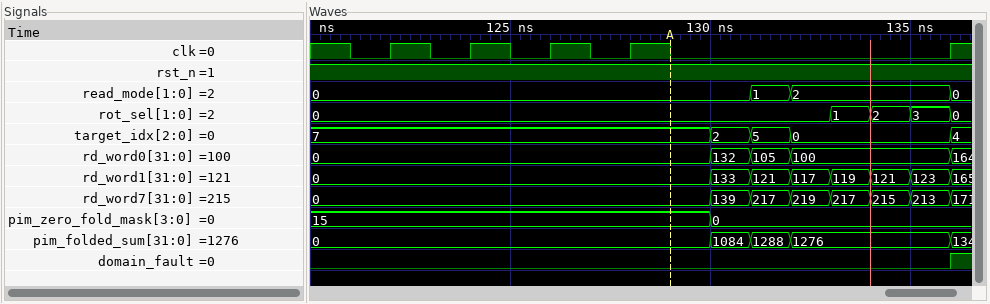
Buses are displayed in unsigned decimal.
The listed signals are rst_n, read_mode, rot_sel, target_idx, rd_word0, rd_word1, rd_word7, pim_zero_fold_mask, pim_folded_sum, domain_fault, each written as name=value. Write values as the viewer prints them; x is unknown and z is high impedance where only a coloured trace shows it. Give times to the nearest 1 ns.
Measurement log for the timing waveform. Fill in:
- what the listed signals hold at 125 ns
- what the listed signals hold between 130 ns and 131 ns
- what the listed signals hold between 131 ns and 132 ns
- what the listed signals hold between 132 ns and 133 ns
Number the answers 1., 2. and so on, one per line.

1. rst_n=1, read_mode=0, rot_sel=0, target_idx=7, rd_word0=0, rd_word1=0, rd_word7=0, pim_zero_fold_mask=15, pim_folded_sum=0, domain_fault=0
2. rst_n=1, read_mode=0, rot_sel=0, target_idx=2, rd_word0=132, rd_word1=133, rd_word7=139, pim_zero_fold_mask=0, pim_folded_sum=1084, domain_fault=0
3. rst_n=1, read_mode=1, rot_sel=0, target_idx=5, rd_word0=105, rd_word1=121, rd_word7=217, pim_zero_fold_mask=0, pim_folded_sum=1288, domain_fault=0
4. rst_n=1, read_mode=2, rot_sel=0, target_idx=0, rd_word0=100, rd_word1=117, rd_word7=219, pim_zero_fold_mask=0, pim_folded_sum=1276, domain_fault=0
